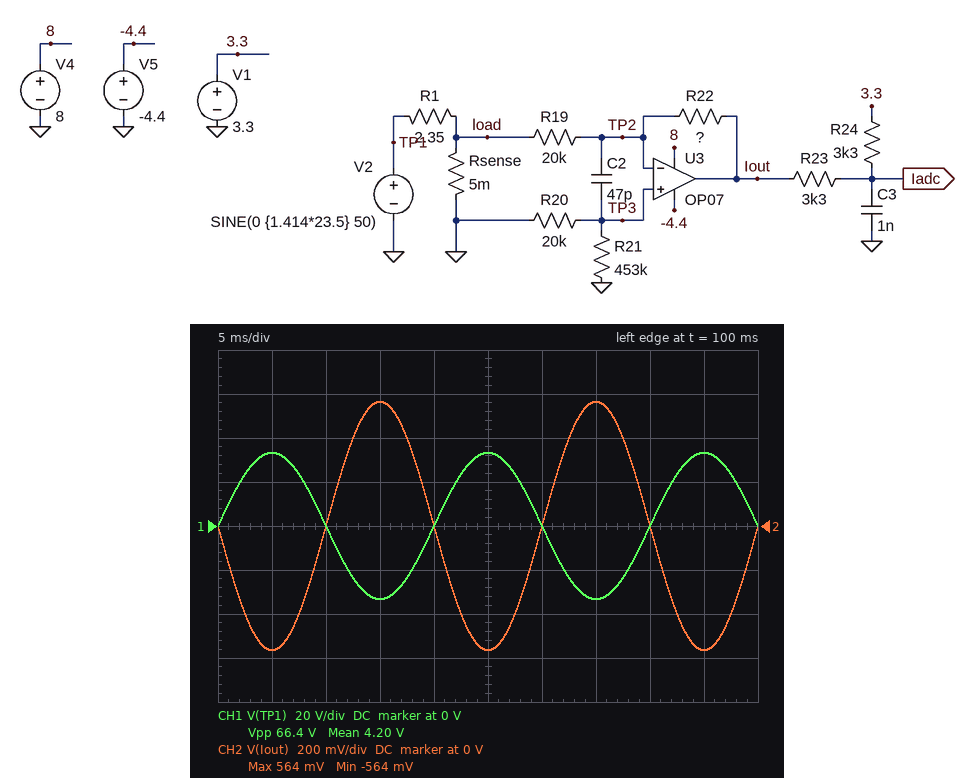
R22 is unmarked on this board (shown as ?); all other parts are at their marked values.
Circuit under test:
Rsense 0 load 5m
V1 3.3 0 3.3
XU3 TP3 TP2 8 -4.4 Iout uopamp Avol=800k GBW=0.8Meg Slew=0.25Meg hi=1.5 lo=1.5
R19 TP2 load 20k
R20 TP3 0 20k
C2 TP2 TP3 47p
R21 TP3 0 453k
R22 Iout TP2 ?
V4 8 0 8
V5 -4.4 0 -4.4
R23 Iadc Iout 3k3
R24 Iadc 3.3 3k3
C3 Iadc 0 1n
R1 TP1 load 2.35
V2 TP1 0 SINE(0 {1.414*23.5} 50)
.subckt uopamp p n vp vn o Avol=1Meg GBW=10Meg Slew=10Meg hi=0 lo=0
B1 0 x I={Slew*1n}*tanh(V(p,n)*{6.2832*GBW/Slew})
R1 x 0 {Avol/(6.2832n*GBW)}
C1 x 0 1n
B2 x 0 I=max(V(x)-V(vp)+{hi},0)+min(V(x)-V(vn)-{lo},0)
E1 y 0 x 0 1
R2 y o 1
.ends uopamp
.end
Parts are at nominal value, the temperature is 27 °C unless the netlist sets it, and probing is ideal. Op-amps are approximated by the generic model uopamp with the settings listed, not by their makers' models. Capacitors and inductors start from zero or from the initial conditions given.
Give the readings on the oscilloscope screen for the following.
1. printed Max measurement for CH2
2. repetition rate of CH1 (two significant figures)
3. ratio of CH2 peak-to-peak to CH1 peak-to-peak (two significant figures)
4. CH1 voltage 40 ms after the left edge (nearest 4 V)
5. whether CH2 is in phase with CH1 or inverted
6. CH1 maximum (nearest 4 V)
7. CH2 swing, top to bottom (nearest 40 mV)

564 mV
50 Hz
0.017
0 V
inverted
32 V
1.12 V
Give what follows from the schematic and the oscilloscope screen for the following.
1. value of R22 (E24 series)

160 kΩ
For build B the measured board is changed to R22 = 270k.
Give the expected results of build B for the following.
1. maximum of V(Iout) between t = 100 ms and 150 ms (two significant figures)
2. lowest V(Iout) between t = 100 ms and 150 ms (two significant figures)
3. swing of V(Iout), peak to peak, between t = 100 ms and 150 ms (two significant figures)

950 mV
-950 mV
1.9 V
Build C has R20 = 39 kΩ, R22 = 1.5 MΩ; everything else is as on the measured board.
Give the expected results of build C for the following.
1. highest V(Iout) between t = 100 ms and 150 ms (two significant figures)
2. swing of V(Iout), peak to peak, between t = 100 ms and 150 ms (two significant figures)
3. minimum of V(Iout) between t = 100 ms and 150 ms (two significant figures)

5.3 V
8.2 V
-2.9 V
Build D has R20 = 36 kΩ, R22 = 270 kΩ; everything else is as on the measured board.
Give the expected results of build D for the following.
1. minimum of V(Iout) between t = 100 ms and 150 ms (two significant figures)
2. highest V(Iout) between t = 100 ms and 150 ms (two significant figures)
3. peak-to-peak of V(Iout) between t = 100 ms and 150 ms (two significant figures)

-950 mV
950 mV
1.9 V
